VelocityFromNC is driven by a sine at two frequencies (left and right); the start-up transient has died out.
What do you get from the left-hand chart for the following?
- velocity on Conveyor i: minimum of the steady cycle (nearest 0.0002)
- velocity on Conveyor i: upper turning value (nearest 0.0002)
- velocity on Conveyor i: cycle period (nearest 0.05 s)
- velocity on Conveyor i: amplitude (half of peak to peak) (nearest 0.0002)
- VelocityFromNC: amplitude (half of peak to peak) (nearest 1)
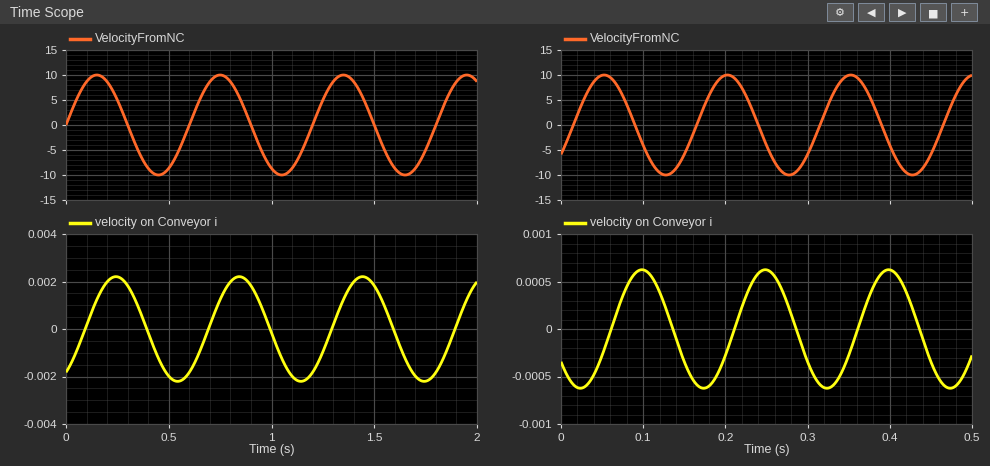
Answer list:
-0.0022
0.0022
0.60 s
0.0022
10
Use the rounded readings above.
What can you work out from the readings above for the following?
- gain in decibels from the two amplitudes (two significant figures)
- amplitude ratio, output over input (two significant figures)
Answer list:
-73 dB
0.00022
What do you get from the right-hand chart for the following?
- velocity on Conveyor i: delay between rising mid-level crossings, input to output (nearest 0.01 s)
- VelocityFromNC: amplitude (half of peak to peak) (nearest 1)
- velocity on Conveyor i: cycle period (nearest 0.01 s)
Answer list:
0.05 s
10
0.15 s
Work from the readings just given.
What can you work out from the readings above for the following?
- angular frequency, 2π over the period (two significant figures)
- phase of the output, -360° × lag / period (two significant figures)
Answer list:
42 rad/s
-120°
